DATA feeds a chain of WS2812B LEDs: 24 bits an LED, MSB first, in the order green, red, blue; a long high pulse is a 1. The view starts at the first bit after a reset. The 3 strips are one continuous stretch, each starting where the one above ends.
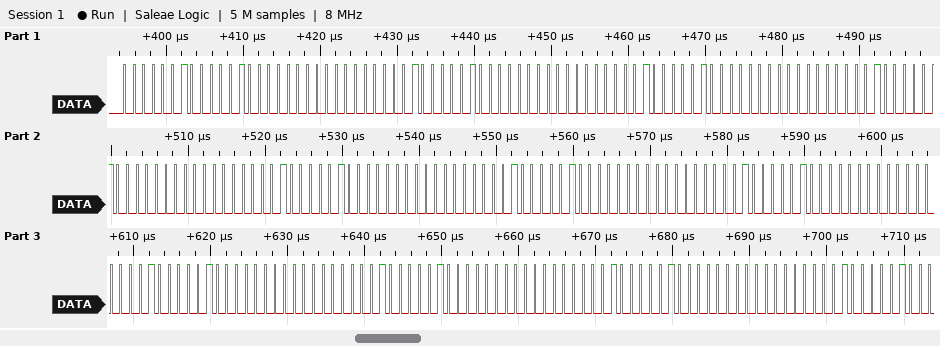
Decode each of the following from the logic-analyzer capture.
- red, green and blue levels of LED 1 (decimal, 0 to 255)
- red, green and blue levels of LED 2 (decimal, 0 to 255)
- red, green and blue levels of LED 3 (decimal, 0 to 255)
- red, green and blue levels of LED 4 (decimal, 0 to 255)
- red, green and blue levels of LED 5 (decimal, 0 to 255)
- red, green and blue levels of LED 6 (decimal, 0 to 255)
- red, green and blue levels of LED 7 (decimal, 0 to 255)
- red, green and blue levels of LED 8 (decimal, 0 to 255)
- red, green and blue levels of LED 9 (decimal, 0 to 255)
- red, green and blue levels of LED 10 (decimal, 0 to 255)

8, 2, 0
8, 2, 0
8, 2, 0
8, 2, 0
8, 2, 0
8, 2, 0
8, 2, 0
8, 2, 0
8, 2, 0
8, 2, 0
